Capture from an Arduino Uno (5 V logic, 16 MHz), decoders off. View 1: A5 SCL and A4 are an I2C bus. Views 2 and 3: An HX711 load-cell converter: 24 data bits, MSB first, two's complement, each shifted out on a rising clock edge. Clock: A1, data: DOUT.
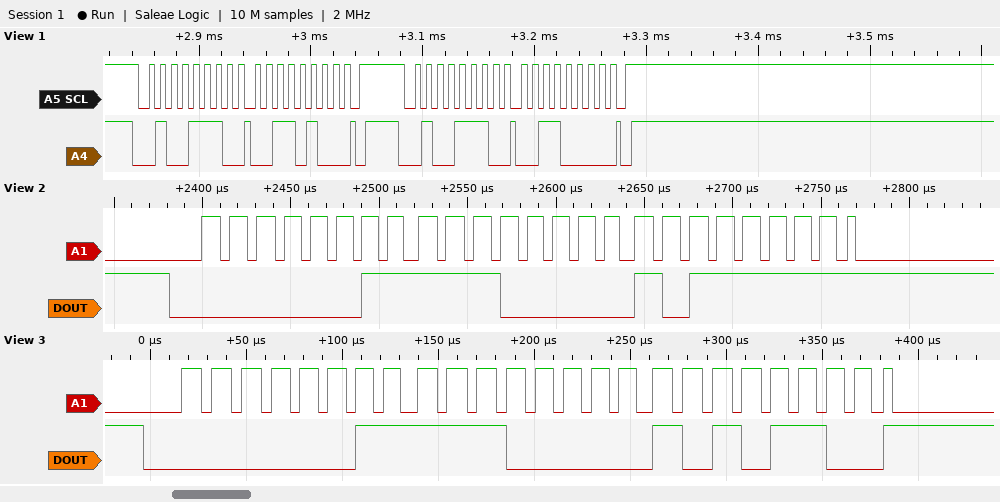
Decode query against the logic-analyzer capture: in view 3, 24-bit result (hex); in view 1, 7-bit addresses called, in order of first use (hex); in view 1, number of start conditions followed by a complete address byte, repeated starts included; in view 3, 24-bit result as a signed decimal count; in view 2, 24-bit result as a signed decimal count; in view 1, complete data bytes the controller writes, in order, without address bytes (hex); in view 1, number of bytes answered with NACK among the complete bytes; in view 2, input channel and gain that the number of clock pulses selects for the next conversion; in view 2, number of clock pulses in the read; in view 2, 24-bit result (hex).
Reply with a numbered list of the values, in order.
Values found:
1. 0x03E0AC
2. 0x27
3. 2
4. 254124
5. 254143
6. 34 30
7. 0
8. channel A, gain 128
9. 25
10. 0x03E0BF
